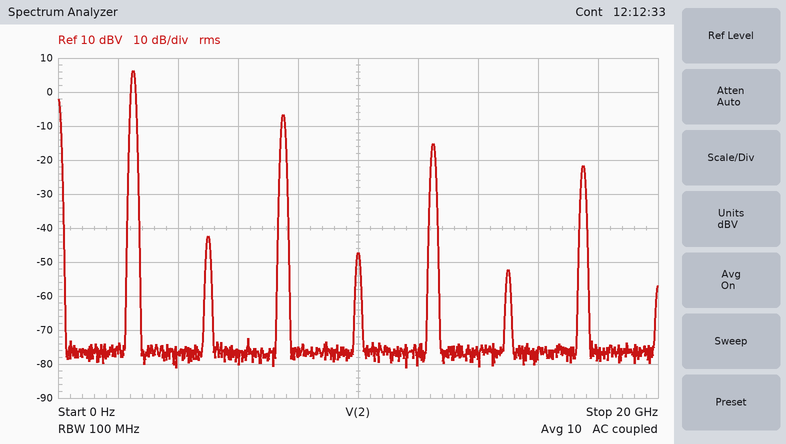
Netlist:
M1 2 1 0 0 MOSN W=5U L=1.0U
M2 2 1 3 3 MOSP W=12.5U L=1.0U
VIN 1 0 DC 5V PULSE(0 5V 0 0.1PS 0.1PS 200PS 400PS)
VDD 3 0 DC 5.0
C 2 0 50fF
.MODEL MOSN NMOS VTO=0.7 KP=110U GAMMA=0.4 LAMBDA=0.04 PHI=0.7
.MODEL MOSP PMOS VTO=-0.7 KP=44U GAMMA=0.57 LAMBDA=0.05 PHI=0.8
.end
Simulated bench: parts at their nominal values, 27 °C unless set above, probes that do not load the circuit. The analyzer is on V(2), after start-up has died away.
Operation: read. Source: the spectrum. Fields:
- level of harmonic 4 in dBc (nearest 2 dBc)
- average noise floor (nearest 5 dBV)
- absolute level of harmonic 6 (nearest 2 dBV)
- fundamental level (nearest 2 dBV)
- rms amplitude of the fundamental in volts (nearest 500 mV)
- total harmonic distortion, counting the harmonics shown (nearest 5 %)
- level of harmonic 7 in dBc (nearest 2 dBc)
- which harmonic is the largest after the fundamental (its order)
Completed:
-54 dBc
-75 dBV
-52 dBV
6 dBV
2.0 V
25 %
-28 dBc
3
